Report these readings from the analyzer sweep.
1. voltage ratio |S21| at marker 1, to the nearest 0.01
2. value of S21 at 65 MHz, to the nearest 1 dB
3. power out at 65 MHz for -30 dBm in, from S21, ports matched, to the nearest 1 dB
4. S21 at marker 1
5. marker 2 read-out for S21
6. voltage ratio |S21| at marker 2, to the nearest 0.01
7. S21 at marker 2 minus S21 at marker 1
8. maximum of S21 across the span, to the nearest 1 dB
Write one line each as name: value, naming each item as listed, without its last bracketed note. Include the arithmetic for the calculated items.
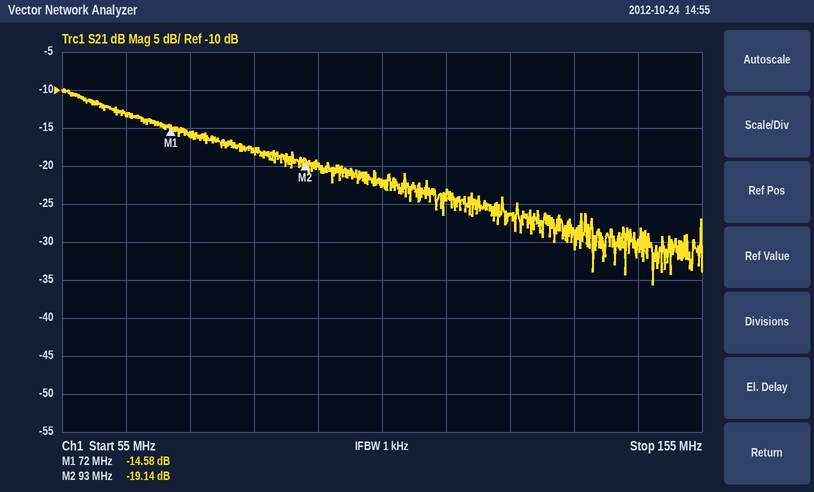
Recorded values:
voltage ratio |S21| at marker 1, to the nearest 0.01: 10^(-14.58/20) ≈ 0.19
value of S21 at 65 MHz, to the nearest 1 dB: -13 dB
power out at 65 MHz for -30 dBm in, from S21, ports matched, to the nearest 1 dB: -30 dBm + (-13 dB) = -43 dBm
S21 at marker 1: -14.58 dB
marker 2 read-out for S21: -19.14 dB
voltage ratio |S21| at marker 2, to the nearest 0.01: 10^(-19.14/20) ≈ 0.11
S21 at marker 2 minus S21 at marker 1: -19.14 − (-14.58) = -4.56 dB
maximum of S21 across the span, to the nearest 1 dB: -10 dB
